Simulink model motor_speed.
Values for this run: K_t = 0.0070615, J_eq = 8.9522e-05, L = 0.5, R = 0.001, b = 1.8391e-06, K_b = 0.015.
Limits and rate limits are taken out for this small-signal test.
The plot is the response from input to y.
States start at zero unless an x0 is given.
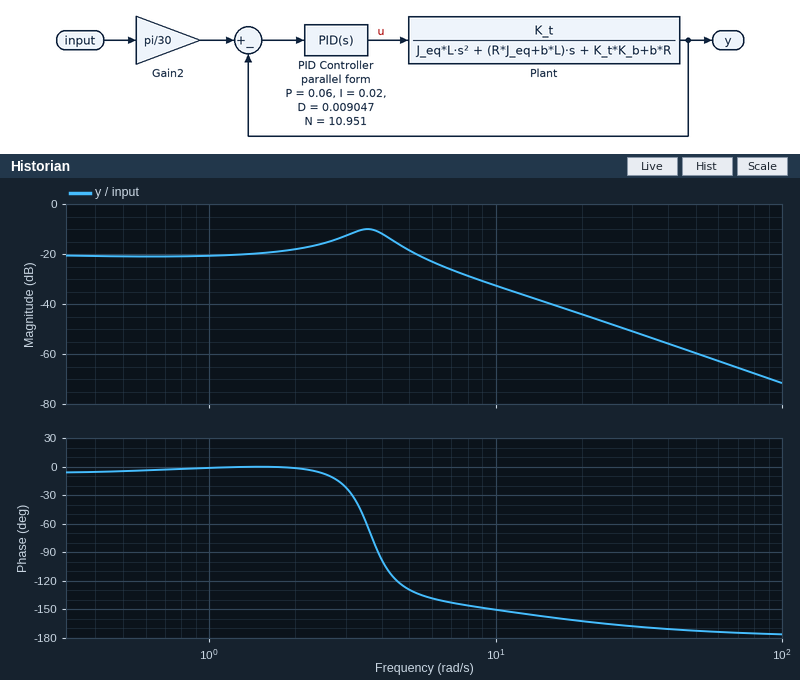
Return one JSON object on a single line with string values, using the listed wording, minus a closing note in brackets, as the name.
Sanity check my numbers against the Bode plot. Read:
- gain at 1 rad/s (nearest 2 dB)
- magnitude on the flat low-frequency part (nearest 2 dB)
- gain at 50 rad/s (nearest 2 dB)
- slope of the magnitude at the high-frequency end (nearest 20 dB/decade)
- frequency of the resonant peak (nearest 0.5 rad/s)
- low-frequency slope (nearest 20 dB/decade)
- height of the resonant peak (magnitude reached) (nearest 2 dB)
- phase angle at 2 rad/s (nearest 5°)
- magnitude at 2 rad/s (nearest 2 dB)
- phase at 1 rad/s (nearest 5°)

{"gain at 1 rad/s": "-20 dB", "magnitude on the flat low-frequency part": "-20 dB", "gain at 50 rad/s": "-60 dB", "slope of the magnitude at the high-frequency end": "-40 dB/decade", "frequency of the resonant peak": "3.5 rad/s", "low-frequency slope": "0 dB/decade", "height of the resonant peak (magnitude reached)": "-10 dB", "phase angle at 2 rad/s": "0°", "magnitude at 2 rad/s": "-18 dB", "phase at 1 rad/s": "0°"}
